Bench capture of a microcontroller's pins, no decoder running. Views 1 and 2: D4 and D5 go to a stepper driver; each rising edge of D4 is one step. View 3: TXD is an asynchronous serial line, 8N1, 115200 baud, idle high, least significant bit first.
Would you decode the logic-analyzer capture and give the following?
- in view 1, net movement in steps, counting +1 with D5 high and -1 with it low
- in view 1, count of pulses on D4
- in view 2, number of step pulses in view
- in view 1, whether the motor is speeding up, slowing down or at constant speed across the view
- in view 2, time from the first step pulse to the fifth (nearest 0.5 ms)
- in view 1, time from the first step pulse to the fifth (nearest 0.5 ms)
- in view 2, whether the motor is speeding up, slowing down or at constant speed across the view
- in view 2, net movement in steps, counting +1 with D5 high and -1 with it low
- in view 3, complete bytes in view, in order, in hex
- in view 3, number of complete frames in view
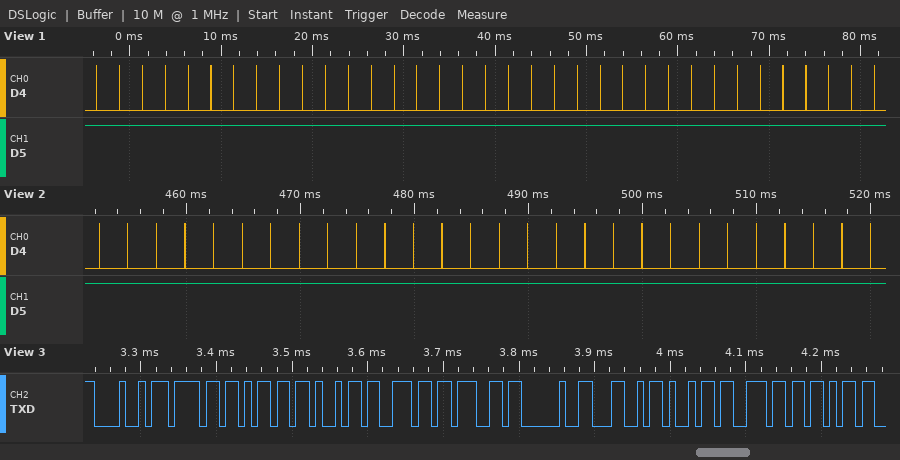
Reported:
+35
35
28
constant speed
10.0 ms
10.0 ms
constant speed
+28
0x48 0x6F 0x6D 0x69 0x6E 0x67 0x20 0x4C 0x69 0x6E 0x6B
11
